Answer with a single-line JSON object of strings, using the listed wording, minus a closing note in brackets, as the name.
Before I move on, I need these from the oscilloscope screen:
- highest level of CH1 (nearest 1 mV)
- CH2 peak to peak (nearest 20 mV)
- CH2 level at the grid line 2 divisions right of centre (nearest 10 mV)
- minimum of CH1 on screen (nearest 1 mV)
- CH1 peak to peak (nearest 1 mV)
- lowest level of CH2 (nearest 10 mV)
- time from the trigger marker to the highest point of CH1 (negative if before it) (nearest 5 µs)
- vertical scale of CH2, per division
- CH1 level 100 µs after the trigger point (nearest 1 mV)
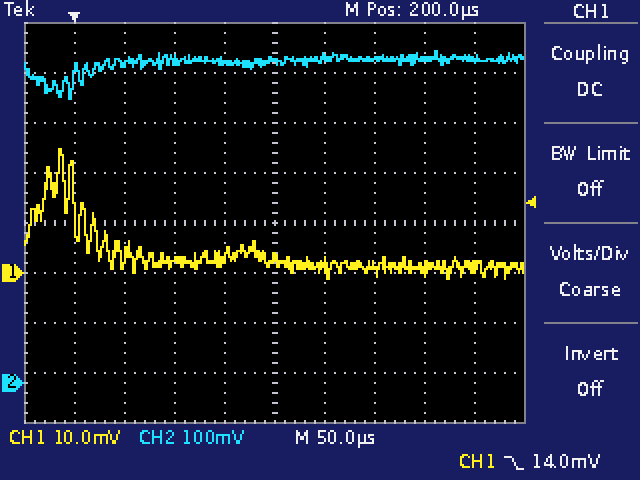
{"highest level of CH1": "25 mV", "CH2 peak to peak": "100 mV", "CH2 level at the grid line 2 divisions right of centre": "650 mV", "minimum of CH1 on screen": "-1 mV", "CH1 peak to peak": "26 mV", "lowest level of CH2": "570 mV", "time from the trigger marker to the highest point of CH1 (negative if before it)": "-15 µs", "vertical scale of CH2, per division": "100 mV", "CH1 level 100 µs after the trigger point": "2 mV"}
